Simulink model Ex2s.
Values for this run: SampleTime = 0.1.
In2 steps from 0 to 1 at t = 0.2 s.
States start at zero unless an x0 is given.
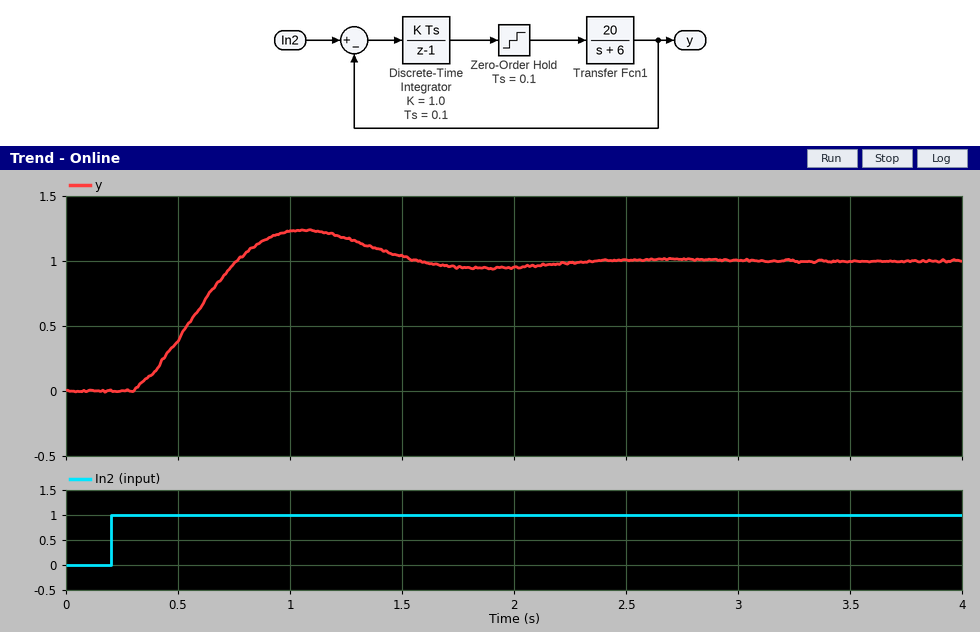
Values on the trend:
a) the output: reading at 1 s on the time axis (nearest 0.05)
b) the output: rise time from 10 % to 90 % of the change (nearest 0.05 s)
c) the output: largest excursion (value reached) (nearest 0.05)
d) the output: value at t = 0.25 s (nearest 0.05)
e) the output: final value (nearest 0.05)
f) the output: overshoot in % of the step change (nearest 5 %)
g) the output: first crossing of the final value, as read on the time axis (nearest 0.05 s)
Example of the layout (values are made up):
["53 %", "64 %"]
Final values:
["1.25", "0.35 s", "1.25", "0.00", "1.00", "25 %", "0.75 s"]
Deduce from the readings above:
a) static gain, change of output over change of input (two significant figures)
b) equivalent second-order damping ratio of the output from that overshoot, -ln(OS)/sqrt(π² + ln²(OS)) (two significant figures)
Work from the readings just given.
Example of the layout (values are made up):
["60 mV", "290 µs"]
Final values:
["1.0", "0.40"]
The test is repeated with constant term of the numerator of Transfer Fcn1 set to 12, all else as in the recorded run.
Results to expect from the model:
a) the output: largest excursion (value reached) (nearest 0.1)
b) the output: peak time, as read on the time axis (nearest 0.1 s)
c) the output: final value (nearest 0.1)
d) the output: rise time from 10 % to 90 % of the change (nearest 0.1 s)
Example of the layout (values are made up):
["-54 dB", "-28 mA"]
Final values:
["1.1", "1.5 s", "1.0", "0.6 s"]
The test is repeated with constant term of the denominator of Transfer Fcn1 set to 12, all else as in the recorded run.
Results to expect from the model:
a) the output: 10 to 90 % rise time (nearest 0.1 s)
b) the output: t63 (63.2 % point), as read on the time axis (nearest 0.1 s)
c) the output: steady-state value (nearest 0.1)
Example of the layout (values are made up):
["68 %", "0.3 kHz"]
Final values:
["0.8 s", "0.8 s", "1.0"]
